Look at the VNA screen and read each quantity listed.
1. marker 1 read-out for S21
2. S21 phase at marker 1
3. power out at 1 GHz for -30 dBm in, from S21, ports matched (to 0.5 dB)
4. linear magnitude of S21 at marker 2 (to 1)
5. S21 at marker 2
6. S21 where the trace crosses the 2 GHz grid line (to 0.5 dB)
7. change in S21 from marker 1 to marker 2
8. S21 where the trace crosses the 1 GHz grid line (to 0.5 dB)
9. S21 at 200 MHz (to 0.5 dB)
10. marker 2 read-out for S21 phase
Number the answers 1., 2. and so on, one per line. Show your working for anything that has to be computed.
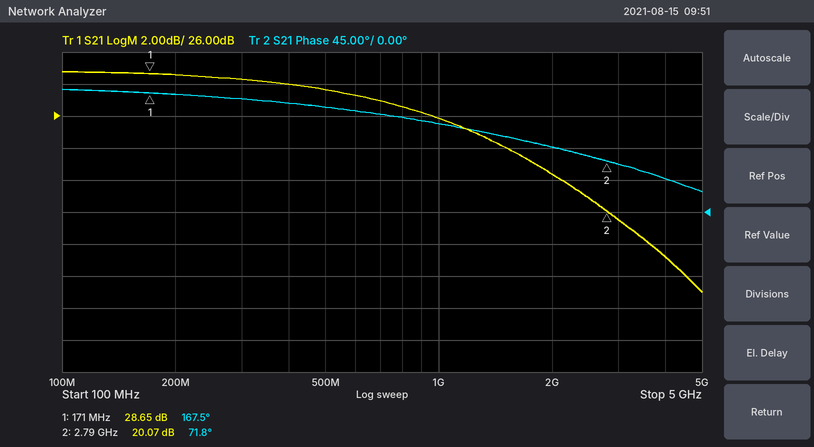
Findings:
1. 28.65 dB
2. 167.5°
3. -30 dBm + (26.0 dB) = -4.0 dBm
4. 10^(20.07/20) ≈ 10
5. 20.07 dB
6. 22.5 dB
7. 20.07 − (28.65) = -8.58 dB
8. 26.0 dB
9. 28.5 dB
10. 71.8°
